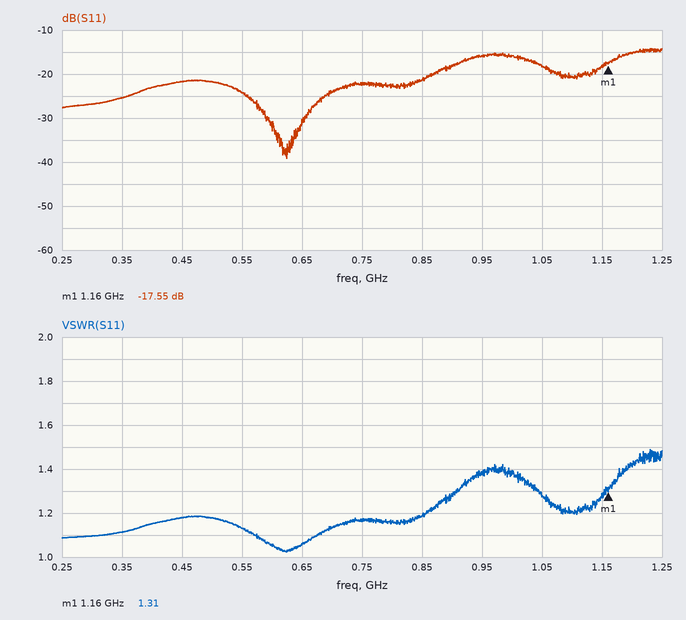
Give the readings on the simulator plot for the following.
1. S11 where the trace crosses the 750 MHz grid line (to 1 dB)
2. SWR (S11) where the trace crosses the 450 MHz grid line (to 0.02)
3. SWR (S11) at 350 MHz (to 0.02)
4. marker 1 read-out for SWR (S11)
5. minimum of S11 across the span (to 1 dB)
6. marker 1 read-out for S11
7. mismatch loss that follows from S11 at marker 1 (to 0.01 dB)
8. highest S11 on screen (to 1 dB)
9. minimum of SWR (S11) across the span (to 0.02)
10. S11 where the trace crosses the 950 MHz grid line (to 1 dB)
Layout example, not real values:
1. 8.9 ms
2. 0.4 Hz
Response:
1. -22 dB
2. 1.18
3. 1.12
4. 1.31
5. -39 dB
6. -17.55 dB
7. 0.08 dB
8. -14 dB
9. 1.02
10. -16 dB
